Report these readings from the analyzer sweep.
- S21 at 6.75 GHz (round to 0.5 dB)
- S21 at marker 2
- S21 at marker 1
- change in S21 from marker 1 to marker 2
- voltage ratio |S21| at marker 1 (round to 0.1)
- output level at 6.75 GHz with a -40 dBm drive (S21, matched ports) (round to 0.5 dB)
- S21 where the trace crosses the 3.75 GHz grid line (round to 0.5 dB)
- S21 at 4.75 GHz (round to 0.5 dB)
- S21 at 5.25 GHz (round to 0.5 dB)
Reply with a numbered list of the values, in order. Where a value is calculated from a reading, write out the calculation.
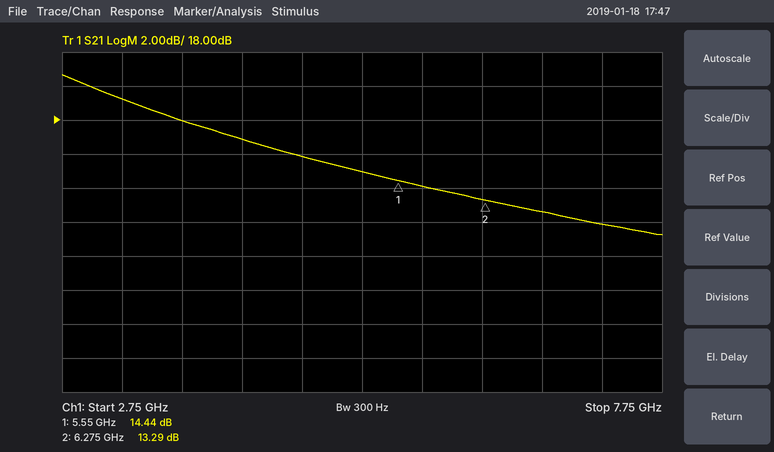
1. 12.5 dB
2. 13.29 dB
3. 14.44 dB
4. 13.29 − (14.44) = -1.15 dB
5. 10^(14.44/20) ≈ 5.3
6. -40 dBm + (12.5 dB) = -27.5 dBm
7. 18.0 dB
8. 16.0 dB
9. 15.0 dB
